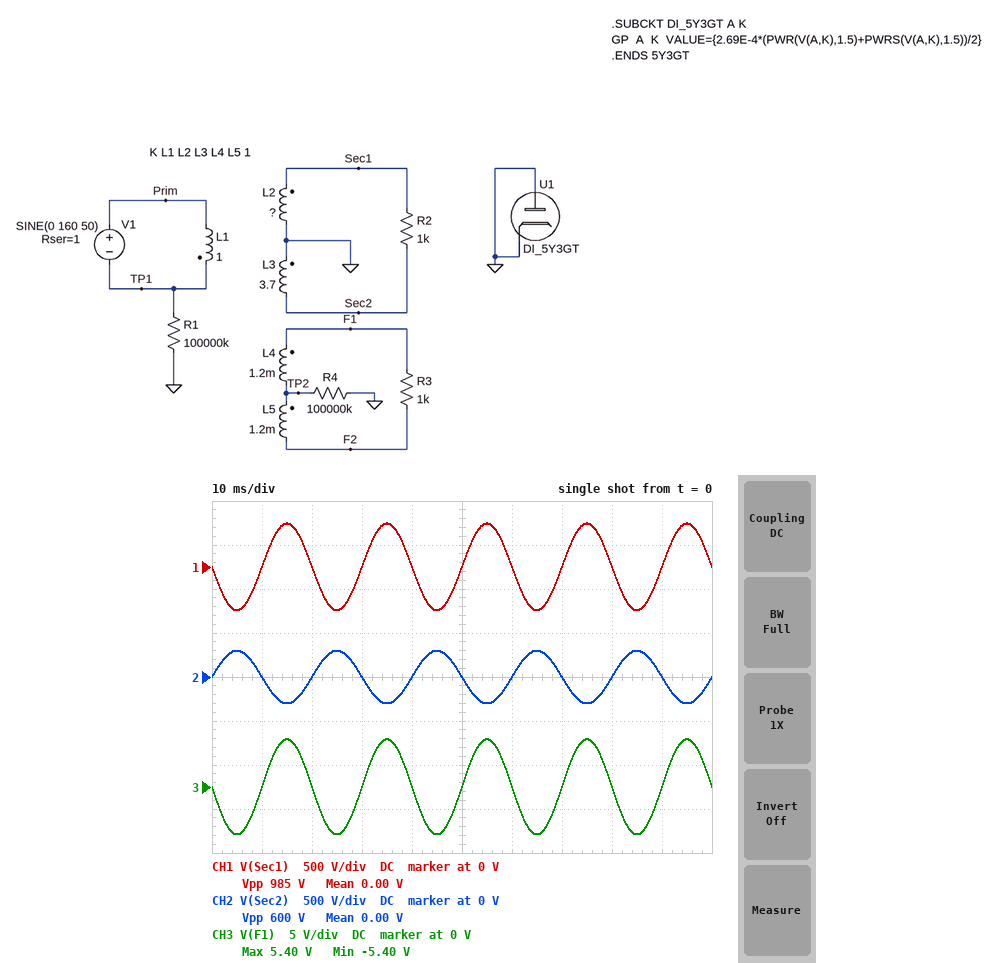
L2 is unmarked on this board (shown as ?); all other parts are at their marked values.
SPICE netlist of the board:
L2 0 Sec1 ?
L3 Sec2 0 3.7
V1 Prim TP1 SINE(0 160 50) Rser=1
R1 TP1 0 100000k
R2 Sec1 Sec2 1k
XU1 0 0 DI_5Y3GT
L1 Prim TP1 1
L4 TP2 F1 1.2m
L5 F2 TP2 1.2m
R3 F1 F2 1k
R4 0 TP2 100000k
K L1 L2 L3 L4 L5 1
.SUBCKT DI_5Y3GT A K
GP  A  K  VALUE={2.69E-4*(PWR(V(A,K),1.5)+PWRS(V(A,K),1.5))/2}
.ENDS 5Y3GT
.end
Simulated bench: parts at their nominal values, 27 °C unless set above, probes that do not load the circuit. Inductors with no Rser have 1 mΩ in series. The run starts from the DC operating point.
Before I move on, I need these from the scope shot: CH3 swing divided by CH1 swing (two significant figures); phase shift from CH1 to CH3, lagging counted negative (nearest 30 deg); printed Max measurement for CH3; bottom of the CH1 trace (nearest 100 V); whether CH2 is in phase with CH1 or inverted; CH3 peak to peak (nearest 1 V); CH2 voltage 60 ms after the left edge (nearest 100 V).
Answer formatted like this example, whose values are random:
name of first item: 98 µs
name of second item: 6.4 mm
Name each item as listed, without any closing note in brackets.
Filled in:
CH3 swing divided by CH1 swing: 0.011
phase shift from CH1 to CH3, lagging counted negative: 0 deg
printed Max measurement for CH3: 5.40 V
bottom of the CH1 trace: -500 V
whether CH2 is in phase with CH1 or inverted: inverted
CH3 peak to peak: 11 V
CH2 voltage 60 ms after the left edge: 0 V
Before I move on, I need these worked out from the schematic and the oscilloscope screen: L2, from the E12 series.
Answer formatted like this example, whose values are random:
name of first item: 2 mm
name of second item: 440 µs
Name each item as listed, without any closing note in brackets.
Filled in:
L2, from the E12 series: 10 H
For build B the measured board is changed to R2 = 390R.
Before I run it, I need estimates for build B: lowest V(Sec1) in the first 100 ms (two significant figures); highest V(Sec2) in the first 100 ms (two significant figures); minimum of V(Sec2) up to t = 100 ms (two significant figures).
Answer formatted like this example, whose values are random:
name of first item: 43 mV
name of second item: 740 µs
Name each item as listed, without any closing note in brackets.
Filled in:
lowest V(Sec1) in the first 100 ms: -470 V
highest V(Sec2) in the first 100 ms: 290 V
minimum of V(Sec2) up to t = 100 ms: -290 V
